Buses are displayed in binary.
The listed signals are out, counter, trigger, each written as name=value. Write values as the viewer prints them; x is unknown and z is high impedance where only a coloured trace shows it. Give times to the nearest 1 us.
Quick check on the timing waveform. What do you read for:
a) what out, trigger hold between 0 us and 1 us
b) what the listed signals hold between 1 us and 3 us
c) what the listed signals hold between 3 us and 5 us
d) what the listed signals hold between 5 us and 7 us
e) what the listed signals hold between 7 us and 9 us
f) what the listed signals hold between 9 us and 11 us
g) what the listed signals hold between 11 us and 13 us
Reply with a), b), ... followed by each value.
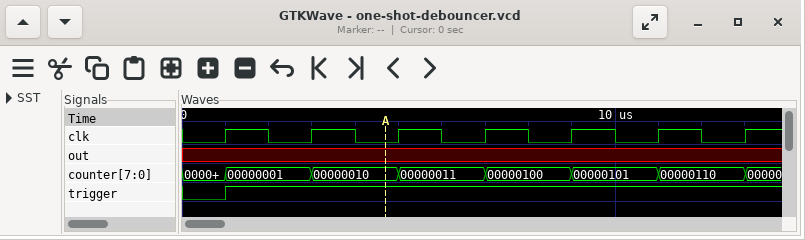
a) out=x, trigger=0
b) out=x, counter=00000001, trigger=1
c) out=x, counter=00000010, trigger=1
d) out=x, counter=00000011, trigger=1
e) out=x, counter=00000100, trigger=1
f) out=x, counter=00000101, trigger=1
g) out=x, counter=00000110, trigger=1
